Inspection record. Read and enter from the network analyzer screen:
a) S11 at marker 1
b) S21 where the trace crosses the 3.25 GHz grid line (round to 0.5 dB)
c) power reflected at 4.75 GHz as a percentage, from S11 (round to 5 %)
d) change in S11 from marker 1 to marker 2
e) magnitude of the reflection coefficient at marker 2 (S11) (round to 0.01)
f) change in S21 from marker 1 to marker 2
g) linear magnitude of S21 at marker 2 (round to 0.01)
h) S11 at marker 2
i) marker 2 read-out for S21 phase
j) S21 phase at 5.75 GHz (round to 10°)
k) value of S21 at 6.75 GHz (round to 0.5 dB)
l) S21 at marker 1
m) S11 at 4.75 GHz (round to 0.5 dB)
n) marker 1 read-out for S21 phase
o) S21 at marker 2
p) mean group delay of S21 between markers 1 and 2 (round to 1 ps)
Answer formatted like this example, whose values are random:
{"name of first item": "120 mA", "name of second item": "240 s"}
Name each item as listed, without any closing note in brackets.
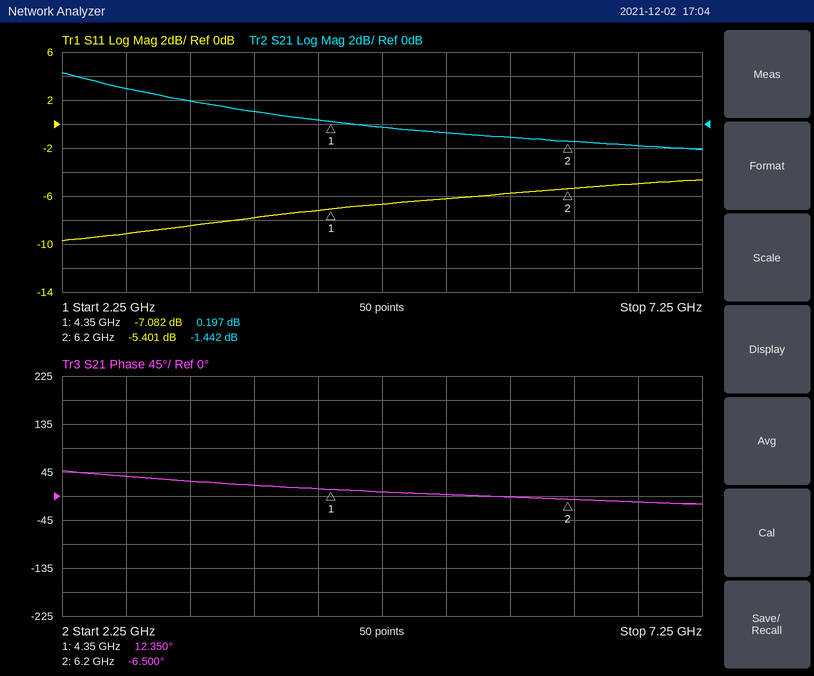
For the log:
{"S11 at marker 1": "-7.082 dB", "S21 where the trace crosses the 3.25 GHz grid line": "2.0 dB", "power reflected at 4.75 GHz as a percentage, from S11": "20 %", "change in S11 from marker 1 to marker 2": "1.681 dB", "magnitude of the reflection coefficient at marker 2 (S11)": "0.54", "change in S21 from marker 1 to marker 2": "-1.639 dB", "linear magnitude of S21 at marker 2": "0.85", "S11 at marker 2": "-5.401 dB", "marker 2 read-out for S21 phase": "-6.500°", "S21 phase at 5.75 GHz": "0°", "value of S21 at 6.75 GHz": "-2.0 dB", "S21 at marker 1": "0.197 dB", "S11 at 4.75 GHz": "-6.5 dB", "marker 1 read-out for S21 phase": "12.350°", "S21 at marker 2": "-1.442 dB", "mean group delay of S21 between markers 1 and 2": "28 ps"}
